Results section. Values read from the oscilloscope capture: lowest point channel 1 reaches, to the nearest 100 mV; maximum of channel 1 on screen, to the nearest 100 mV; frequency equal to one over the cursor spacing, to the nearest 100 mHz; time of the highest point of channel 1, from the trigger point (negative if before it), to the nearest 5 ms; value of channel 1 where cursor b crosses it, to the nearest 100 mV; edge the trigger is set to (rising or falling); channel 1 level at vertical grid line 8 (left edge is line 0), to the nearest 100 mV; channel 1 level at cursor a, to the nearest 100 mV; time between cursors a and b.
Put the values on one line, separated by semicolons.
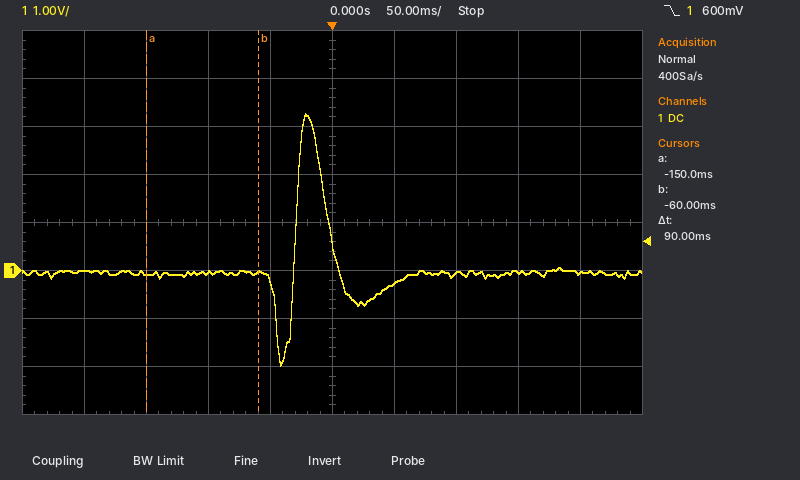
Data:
-2.0 V; 3.3 V; 11.1 Hz; -20 ms; 0.0 V; falling; 0.0 V; -100 mV; 90 ms
